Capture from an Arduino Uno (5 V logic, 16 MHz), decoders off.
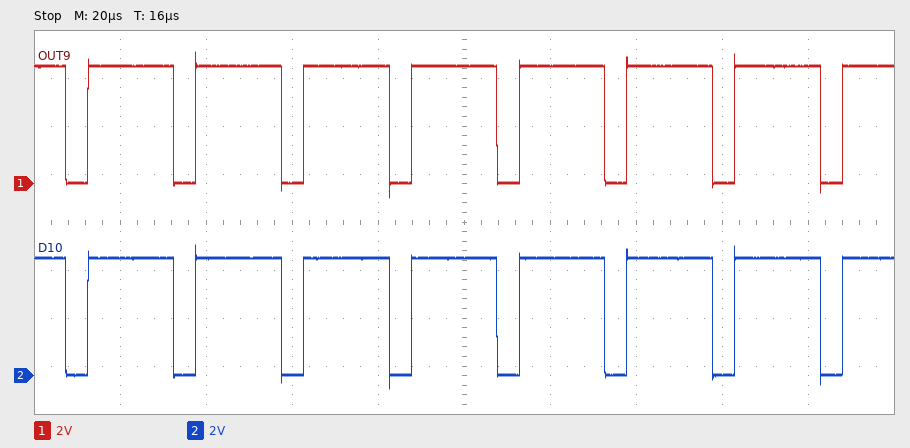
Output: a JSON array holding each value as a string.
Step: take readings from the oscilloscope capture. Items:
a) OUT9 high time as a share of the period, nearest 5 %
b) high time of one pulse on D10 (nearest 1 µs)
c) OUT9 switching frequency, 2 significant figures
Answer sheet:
["80 %", "20 µs", "40 kHz"]
